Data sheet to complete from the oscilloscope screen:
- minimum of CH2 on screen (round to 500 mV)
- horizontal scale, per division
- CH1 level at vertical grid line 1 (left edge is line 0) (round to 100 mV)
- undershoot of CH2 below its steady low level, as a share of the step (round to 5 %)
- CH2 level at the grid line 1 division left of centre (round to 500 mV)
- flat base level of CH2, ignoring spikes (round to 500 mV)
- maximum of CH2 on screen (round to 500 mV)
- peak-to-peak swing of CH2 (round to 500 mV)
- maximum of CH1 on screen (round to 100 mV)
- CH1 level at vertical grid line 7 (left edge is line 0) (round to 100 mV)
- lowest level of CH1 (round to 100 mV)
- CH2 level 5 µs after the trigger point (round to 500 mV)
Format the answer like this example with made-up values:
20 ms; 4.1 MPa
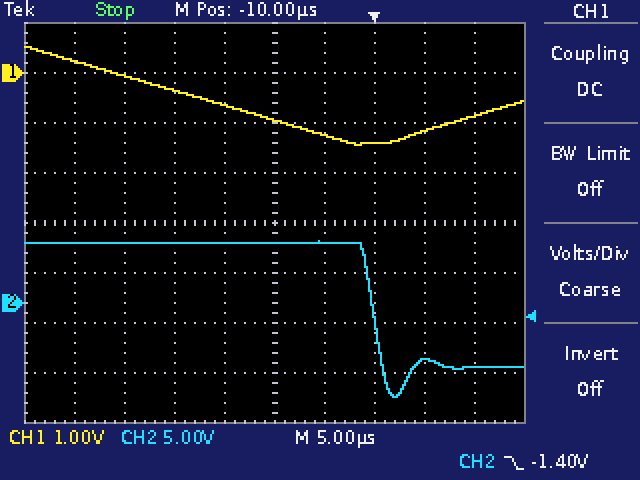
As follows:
-9.5 V; 5 µs; 200 mV; 25 %; 6.0 V; -6.5 V; 6.0 V; 15.5 V; 500 mV; -1.4 V; -1.4 V; -5.5 V
